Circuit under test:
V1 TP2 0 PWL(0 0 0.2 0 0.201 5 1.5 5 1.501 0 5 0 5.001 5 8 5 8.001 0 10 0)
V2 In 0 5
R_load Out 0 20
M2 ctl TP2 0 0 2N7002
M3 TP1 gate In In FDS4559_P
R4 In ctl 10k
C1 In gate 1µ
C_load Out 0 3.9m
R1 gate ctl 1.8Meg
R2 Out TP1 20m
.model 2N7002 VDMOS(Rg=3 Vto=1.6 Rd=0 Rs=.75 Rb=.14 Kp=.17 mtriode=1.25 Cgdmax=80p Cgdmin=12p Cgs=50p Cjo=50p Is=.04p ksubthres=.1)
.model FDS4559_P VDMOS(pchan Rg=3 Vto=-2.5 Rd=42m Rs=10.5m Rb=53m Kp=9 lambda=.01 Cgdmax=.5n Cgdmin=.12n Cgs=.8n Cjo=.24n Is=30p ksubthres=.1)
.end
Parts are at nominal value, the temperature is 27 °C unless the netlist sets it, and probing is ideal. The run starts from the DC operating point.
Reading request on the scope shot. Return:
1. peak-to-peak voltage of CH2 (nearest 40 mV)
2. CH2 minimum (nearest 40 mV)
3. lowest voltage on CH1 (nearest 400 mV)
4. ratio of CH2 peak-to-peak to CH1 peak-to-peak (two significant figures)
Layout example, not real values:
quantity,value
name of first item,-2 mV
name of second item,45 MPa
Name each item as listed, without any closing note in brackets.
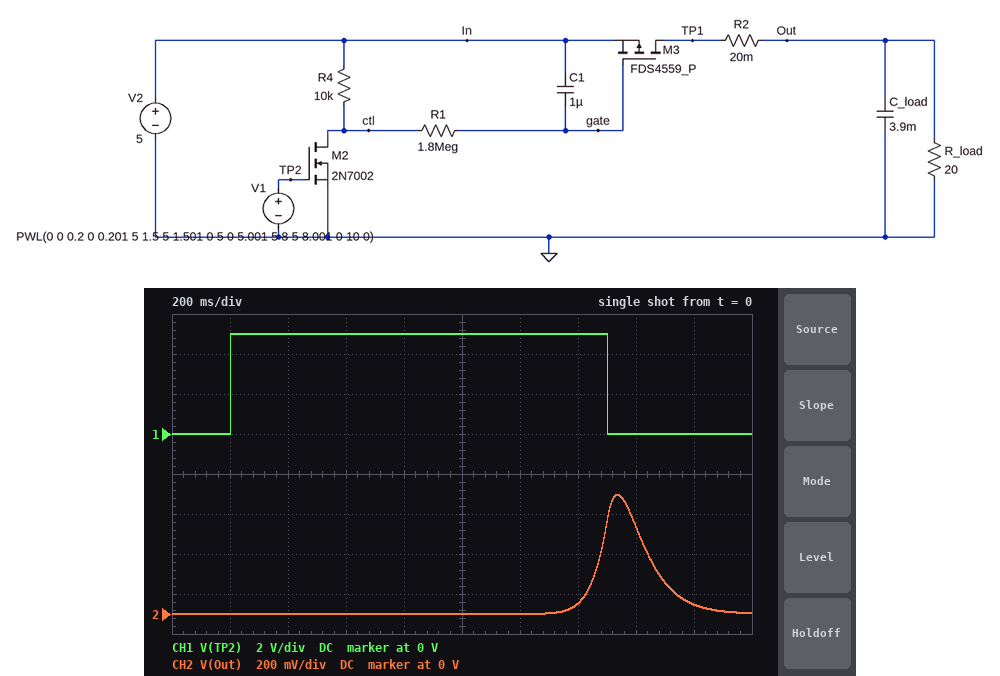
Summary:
quantity,value
peak-to-peak voltage of CH2,600 mV
CH2 minimum,0 V
lowest voltage on CH1,0 V
ratio of CH2 peak-to-peak to CH1 peak-to-peak,0.12
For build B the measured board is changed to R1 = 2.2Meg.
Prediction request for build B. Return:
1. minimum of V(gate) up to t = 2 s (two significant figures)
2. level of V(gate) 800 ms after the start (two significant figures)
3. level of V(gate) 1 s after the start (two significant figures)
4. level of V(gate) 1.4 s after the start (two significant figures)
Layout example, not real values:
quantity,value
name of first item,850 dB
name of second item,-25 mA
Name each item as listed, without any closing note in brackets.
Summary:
quantity,value
minimum of V(gate) up to t = 2 s,2.8 V
level of V(gate) 800 ms after the start,3.8 V
level of V(gate) 1 s after the start,3.5 V
level of V(gate) 1.4 s after the start,2.9 V
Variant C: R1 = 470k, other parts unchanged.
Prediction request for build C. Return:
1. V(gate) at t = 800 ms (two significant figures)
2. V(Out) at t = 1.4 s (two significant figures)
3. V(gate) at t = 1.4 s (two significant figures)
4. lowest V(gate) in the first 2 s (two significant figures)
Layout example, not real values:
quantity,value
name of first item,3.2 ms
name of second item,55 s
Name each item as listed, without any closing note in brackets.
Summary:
quantity,value
V(gate) at t = 800 ms,1.4 V
V(Out) at t = 1.4 s,5.0 V
V(gate) at t = 1.4 s,390 mV
lowest V(gate) in the first 2 s,320 mV
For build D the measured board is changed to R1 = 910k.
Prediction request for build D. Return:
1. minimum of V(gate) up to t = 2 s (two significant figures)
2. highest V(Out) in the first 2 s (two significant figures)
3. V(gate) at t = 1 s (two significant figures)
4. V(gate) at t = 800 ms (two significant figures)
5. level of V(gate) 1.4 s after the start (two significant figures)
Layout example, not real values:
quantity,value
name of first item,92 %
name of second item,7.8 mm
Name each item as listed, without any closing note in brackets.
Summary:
quantity,value
minimum of V(gate) up to t = 2 s,1.2 V
highest V(Out) in the first 2 s,5.0 V
V(gate) at t = 1 s,2.1 V
V(gate) at t = 800 ms,2.6 V
level of V(gate) 1.4 s after the start,1.3 V
